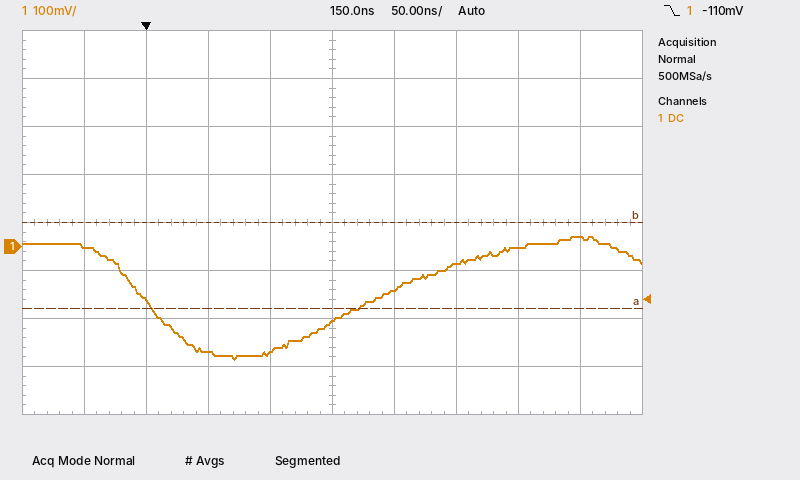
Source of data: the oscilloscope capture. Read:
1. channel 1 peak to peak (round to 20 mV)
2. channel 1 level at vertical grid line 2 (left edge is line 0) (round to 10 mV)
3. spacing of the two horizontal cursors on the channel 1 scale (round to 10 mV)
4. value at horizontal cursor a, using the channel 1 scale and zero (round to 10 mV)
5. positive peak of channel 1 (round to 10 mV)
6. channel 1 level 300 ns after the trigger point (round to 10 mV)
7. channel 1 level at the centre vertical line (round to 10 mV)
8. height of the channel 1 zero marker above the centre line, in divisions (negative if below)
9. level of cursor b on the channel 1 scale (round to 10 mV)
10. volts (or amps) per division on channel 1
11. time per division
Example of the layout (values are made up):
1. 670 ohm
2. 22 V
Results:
1. 260 mV
2. -110 mV
3. 180 mV
4. -130 mV
5. 20 mV
6. 0 mV
7. -160 mV
8. -0.5 div
9. 50 mV
10. 100 mV
11. 50 ns
